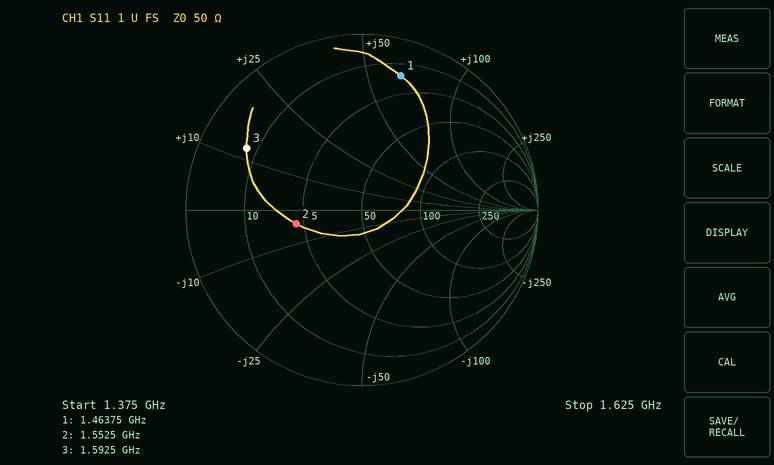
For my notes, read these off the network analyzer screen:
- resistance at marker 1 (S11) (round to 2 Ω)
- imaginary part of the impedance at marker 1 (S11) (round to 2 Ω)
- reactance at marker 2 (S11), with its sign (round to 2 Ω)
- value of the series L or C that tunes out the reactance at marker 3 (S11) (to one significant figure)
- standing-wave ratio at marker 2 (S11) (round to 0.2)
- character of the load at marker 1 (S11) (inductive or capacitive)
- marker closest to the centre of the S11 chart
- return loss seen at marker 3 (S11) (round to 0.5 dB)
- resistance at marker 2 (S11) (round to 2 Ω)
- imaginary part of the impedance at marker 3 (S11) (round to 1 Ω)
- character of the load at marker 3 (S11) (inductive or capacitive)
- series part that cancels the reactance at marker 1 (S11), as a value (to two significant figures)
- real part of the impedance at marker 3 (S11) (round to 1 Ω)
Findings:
16 Ω
+64 Ω
-4 Ω
8 pF
2.2
inductive
marker 2
2.5 dB
22 Ω
+12 Ω
inductive
1.7 pF
8 Ω
